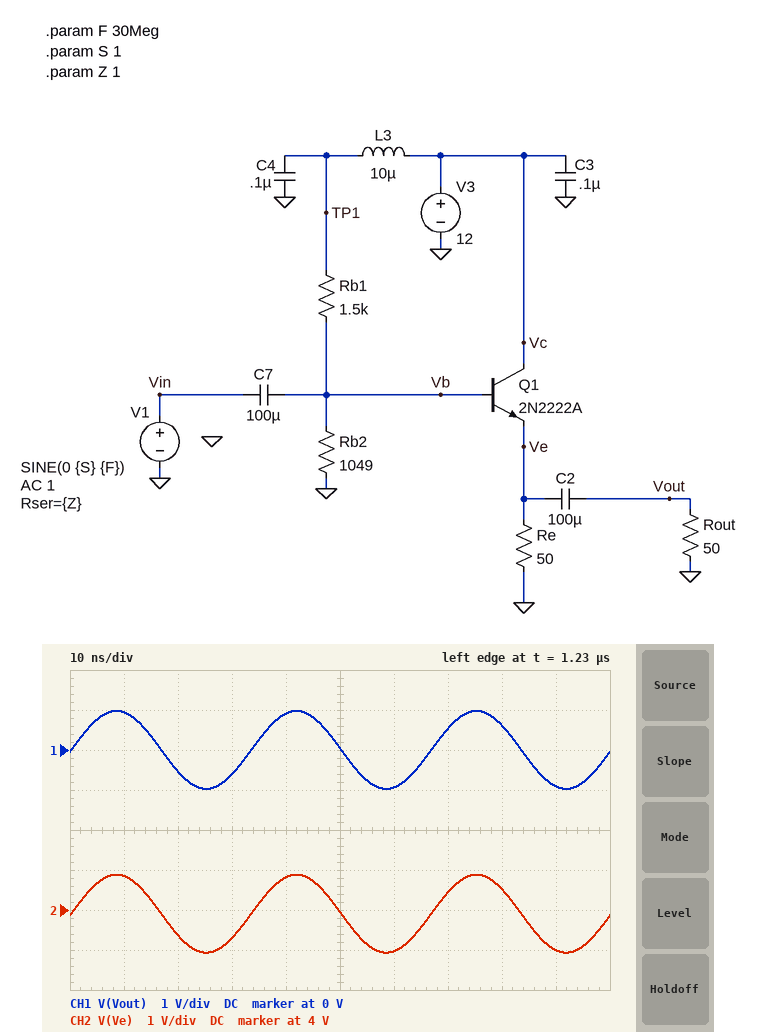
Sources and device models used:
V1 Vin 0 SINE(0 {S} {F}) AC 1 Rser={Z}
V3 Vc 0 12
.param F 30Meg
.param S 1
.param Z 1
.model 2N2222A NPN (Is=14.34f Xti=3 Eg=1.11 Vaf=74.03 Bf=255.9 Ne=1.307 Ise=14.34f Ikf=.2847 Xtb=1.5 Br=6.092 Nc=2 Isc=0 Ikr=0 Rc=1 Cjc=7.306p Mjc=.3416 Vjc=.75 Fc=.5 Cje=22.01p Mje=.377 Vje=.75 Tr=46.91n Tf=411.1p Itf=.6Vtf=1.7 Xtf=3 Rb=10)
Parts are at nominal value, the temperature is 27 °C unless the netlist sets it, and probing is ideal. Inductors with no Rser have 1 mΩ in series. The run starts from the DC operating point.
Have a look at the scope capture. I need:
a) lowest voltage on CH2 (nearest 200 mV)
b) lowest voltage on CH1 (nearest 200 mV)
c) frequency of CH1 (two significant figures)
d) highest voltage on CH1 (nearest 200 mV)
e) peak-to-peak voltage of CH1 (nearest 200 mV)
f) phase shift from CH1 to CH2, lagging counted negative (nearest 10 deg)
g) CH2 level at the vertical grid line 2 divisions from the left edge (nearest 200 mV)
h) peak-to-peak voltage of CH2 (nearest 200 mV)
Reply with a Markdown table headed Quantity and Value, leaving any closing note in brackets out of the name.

| Quantity | Value |
|---|---|
| lowest voltage on CH2 | 3.0 V |
| lowest voltage on CH1 | -1.0 V |
| frequency of CH1 | 30 MHz |
| highest voltage on CH1 | 1.0 V |
| peak-to-peak voltage of CH1 | 2.0 V |
| phase shift from CH1 to CH2, lagging counted negative | 0 deg |
| CH2 level at the vertical grid line 2 divisions from the left edge | 3.4 V |
| peak-to-peak voltage of CH2 | 2.0 V |
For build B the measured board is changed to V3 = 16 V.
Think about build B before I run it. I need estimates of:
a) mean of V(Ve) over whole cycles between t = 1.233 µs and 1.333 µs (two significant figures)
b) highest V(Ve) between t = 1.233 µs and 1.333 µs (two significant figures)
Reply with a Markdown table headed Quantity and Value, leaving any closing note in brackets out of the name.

| Quantity | Value |
|---|---|
| mean of V(Ve) over whole cycles between t = 1.233 µs and 1.333 µs | 5.4 V |
| highest V(Ve) between t = 1.233 µs and 1.333 µs | 6.4 V |
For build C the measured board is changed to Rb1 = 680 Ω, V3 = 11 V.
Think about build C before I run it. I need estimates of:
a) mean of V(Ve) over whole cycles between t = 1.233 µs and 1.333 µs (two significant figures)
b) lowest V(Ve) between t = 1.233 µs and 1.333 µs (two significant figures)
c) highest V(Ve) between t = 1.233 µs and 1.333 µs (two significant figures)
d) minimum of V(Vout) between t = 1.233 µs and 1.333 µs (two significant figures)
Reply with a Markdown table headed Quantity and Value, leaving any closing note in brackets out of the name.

| Quantity | Value |
|---|---|
| mean of V(Ve) over whole cycles between t = 1.233 µs and 1.333 µs | 5.6 V |
| lowest V(Ve) between t = 1.233 µs and 1.333 µs | 4.6 V |
| highest V(Ve) between t = 1.233 µs and 1.333 µs | 6.6 V |
| minimum of V(Vout) between t = 1.233 µs and 1.333 µs | -980 mV |
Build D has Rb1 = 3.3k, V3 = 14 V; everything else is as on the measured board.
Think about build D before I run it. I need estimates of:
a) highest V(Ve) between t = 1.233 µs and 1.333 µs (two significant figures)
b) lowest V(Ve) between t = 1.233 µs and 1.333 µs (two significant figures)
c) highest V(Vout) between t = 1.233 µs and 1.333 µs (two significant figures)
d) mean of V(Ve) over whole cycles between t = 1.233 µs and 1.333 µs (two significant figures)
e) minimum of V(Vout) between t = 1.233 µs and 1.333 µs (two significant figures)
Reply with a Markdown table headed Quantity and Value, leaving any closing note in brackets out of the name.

| Quantity | Value |
|---|---|
| highest V(Ve) between t = 1.233 µs and 1.333 µs | 3.4 V |
| lowest V(Ve) between t = 1.233 µs and 1.333 µs | 1.5 V |
| highest V(Vout) between t = 1.233 µs and 1.333 µs | 970 mV |
| mean of V(Ve) over whole cycles between t = 1.233 µs and 1.333 µs | 2.4 V |
| minimum of V(Vout) between t = 1.233 µs and 1.333 µs | -950 mV |
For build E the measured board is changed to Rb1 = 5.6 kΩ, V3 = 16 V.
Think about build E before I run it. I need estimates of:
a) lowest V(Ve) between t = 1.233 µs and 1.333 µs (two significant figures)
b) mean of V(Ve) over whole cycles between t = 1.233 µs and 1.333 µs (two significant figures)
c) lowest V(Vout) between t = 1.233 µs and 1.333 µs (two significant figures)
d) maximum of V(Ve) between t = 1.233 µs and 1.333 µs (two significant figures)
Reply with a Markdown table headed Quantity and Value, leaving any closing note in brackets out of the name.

| Quantity | Value |
|---|---|
| lowest V(Ve) between t = 1.233 µs and 1.333 µs | 800 mV |
| mean of V(Ve) over whole cycles between t = 1.233 µs and 1.333 µs | 1.7 V |
| lowest V(Vout) between t = 1.233 µs and 1.333 µs | -850 mV |
| maximum of V(Ve) between t = 1.233 µs and 1.333 µs | 2.6 V |
